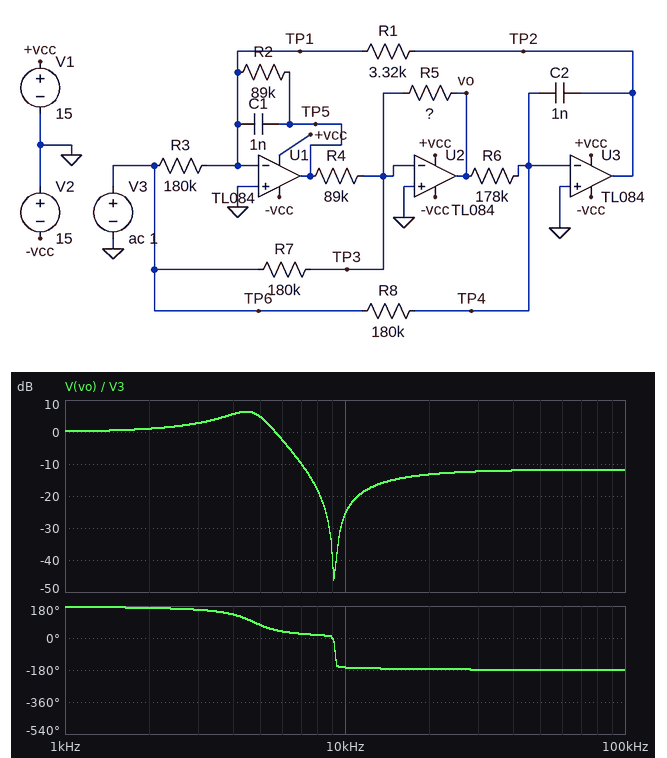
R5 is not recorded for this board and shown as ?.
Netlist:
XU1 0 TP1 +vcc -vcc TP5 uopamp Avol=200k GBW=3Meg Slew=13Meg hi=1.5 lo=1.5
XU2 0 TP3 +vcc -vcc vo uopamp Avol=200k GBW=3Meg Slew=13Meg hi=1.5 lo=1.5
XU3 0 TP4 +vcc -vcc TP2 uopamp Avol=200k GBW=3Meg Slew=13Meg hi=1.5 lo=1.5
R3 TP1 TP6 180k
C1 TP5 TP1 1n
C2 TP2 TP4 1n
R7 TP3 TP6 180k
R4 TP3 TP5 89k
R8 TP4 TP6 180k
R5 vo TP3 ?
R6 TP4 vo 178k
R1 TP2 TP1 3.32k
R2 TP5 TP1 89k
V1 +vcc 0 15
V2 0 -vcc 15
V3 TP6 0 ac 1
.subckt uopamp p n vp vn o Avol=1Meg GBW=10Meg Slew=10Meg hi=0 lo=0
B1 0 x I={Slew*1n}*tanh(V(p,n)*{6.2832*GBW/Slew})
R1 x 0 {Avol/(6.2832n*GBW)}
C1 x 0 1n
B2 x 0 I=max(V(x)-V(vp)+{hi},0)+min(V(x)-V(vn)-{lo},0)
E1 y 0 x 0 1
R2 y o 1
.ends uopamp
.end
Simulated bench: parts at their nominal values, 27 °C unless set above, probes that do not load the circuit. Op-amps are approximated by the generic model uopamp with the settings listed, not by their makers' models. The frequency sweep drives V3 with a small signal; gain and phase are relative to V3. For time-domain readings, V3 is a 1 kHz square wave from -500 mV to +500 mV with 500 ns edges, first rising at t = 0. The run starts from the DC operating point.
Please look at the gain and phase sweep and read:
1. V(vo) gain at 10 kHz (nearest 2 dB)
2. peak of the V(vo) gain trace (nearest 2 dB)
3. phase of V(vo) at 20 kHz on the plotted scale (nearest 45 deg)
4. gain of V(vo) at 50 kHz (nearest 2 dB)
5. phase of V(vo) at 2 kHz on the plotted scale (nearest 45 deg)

-26 dB
6 dB
-180 deg
-12 dB
180 deg
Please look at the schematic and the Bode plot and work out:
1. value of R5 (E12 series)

47 kΩ
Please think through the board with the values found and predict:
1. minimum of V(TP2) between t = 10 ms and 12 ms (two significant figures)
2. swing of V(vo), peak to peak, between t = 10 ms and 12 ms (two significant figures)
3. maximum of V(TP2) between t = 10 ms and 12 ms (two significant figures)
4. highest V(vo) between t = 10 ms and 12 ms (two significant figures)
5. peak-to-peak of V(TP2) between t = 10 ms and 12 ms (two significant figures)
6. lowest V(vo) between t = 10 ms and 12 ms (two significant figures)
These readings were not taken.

-140 mV
1.8 V
140 mV
910 mV
270 mV
-910 mV
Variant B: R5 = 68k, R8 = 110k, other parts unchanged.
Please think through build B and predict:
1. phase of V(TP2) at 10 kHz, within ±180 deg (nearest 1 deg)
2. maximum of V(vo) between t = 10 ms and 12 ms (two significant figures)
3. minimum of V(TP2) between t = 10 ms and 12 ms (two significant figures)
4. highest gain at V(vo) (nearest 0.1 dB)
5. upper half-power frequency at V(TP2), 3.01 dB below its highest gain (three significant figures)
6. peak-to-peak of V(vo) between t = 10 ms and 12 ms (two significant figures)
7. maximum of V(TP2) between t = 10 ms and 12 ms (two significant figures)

91 deg
1.6 V
-190 mV
12.5 dB
6.56 kHz
3.1 V
190 mV
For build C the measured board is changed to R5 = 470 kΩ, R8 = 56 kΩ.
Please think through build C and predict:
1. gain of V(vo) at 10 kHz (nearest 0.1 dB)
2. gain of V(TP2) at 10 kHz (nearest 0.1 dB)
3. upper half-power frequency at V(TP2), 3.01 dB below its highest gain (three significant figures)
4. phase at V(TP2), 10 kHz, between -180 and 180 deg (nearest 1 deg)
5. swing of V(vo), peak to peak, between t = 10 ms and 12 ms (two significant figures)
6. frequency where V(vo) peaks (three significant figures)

11.2 dB
-25.3 dB
15.4 kHz
-135 deg
4.5 V
14.7 kHz
